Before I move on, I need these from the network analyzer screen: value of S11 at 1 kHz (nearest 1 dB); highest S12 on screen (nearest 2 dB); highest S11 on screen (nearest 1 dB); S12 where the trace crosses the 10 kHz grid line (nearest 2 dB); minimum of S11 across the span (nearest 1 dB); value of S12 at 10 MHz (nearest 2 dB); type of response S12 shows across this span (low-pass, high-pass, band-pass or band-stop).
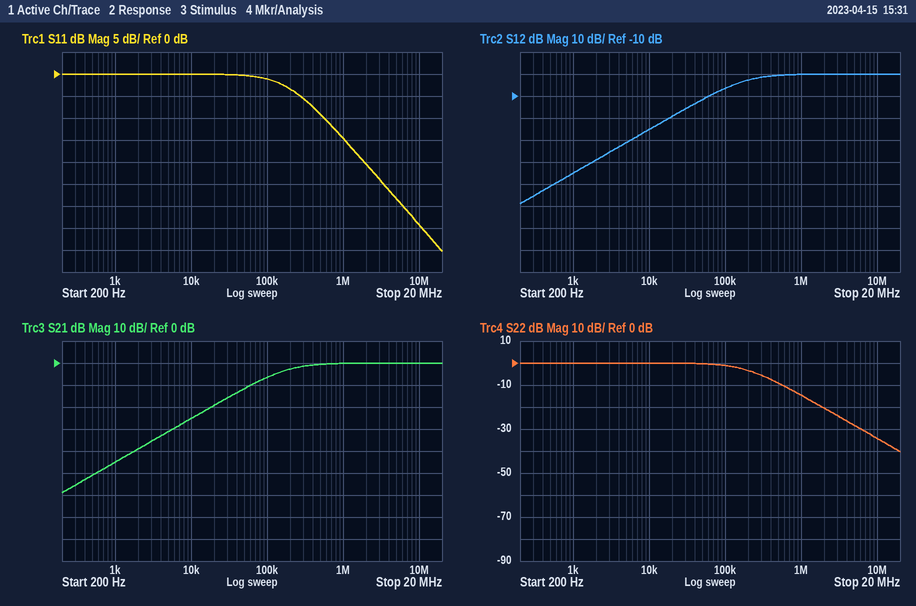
0 dB
0 dB
0 dB
-26 dB
-40 dB
0 dB
high-pass
